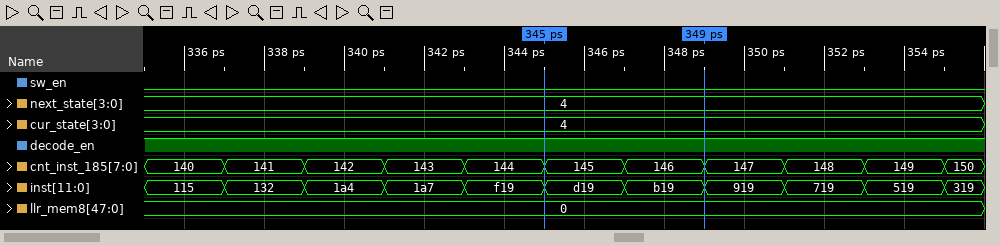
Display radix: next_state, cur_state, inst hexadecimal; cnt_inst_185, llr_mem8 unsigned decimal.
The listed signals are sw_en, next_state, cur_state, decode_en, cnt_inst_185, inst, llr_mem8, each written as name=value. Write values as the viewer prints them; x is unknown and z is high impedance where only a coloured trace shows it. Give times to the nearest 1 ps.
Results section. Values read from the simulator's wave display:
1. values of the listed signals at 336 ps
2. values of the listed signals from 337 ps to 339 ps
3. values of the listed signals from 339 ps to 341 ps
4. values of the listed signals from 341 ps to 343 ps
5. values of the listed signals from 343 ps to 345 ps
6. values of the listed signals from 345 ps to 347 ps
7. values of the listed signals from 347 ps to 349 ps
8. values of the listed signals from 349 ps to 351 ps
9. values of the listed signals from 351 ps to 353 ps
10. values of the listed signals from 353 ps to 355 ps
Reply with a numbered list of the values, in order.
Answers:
1. sw_en=0, next_state=4, cur_state=4, decode_en=1, cnt_inst_185=140, inst=115, llr_mem8=0
2. sw_en=0, next_state=4, cur_state=4, decode_en=1, cnt_inst_185=141, inst=132, llr_mem8=0
3. sw_en=0, next_state=4, cur_state=4, decode_en=1, cnt_inst_185=142, inst=1a4, llr_mem8=0
4. sw_en=0, next_state=4, cur_state=4, decode_en=1, cnt_inst_185=143, inst=1a7, llr_mem8=0
5. sw_en=0, next_state=4, cur_state=4, decode_en=1, cnt_inst_185=144, inst=f19, llr_mem8=0
6. sw_en=0, next_state=4, cur_state=4, decode_en=1, cnt_inst_185=145, inst=d19, llr_mem8=0
7. sw_en=0, next_state=4, cur_state=4, decode_en=1, cnt_inst_185=146, inst=b19, llr_mem8=0
8. sw_en=0, next_state=4, cur_state=4, decode_en=1, cnt_inst_185=147, inst=919, llr_mem8=0
9. sw_en=0, next_state=4, cur_state=4, decode_en=1, cnt_inst_185=148, inst=719, llr_mem8=0
10. sw_en=0, next_state=4, cur_state=4, decode_en=1, cnt_inst_185=149, inst=519, llr_mem8=0
